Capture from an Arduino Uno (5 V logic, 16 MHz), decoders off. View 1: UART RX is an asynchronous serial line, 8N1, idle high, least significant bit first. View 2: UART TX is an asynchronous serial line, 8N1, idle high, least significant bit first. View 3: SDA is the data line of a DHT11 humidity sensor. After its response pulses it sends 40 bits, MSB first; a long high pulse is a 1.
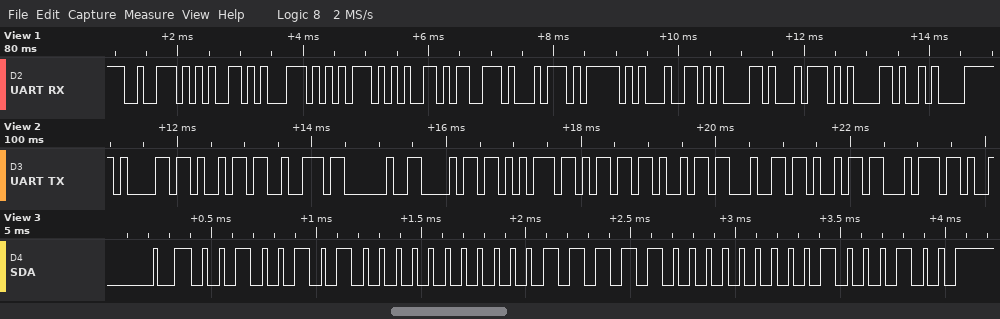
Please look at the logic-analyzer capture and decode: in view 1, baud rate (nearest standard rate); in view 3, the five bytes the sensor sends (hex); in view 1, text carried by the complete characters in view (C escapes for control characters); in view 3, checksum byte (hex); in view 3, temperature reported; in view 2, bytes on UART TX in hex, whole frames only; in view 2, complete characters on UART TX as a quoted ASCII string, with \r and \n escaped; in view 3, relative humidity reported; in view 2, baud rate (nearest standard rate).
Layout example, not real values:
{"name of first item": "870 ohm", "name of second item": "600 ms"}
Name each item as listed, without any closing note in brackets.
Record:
{"in view 1, baud rate": "9600 baud", "in view 3, the five bytes the sensor sends": "25 00 1F 00 44", "in view 1, text carried by the complete characters in view": "\"request_data\\n\"", "in view 3, checksum byte": "0x44", "in view 3, temperature reported": "31.0 °C", "in view 2, bytes on UART TX in hex, whole frames only": "61 69 72 20 68 75 6D 69 64 69 74", "in view 2, complete characters on UART TX as a quoted ASCII string, with \\r and \\n escaped": "\"air humidit\"", "in view 3, relative humidity reported": "37 %", "in view 2, baud rate": "9600 baud"}
